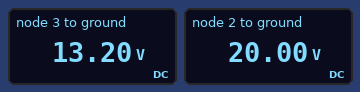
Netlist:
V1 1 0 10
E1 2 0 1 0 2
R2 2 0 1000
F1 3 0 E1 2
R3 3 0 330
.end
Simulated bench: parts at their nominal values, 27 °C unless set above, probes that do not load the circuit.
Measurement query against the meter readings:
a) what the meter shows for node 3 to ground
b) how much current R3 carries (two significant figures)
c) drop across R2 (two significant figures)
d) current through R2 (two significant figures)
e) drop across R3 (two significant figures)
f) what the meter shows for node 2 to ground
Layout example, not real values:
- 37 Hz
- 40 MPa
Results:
- 13.20 V
- 40 mA
- 20 V
- 20 mA
- 13 V
- 20.00 V
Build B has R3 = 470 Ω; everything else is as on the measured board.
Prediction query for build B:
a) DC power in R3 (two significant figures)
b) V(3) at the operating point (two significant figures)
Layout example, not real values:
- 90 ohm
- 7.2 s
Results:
- 750 mW
- 19 V
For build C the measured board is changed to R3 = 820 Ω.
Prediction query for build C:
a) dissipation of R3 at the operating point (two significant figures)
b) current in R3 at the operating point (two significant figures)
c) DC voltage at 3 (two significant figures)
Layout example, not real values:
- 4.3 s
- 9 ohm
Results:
- 1.3 W
- 40 mA
- 33 V
